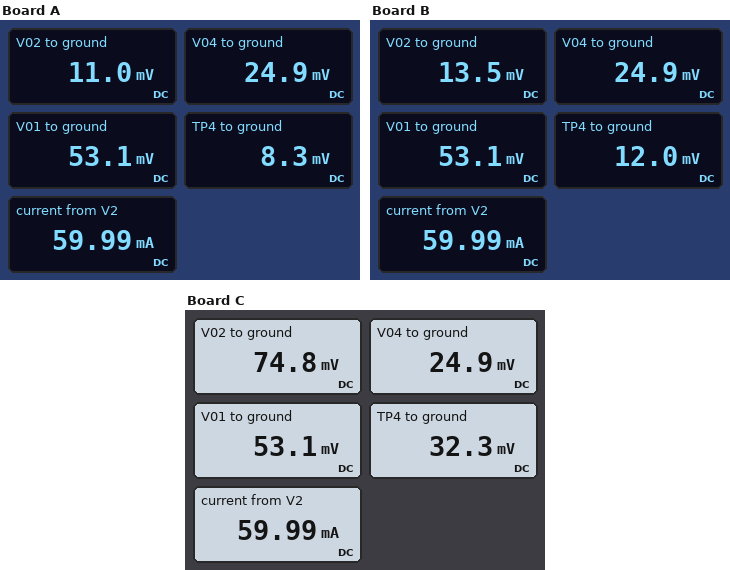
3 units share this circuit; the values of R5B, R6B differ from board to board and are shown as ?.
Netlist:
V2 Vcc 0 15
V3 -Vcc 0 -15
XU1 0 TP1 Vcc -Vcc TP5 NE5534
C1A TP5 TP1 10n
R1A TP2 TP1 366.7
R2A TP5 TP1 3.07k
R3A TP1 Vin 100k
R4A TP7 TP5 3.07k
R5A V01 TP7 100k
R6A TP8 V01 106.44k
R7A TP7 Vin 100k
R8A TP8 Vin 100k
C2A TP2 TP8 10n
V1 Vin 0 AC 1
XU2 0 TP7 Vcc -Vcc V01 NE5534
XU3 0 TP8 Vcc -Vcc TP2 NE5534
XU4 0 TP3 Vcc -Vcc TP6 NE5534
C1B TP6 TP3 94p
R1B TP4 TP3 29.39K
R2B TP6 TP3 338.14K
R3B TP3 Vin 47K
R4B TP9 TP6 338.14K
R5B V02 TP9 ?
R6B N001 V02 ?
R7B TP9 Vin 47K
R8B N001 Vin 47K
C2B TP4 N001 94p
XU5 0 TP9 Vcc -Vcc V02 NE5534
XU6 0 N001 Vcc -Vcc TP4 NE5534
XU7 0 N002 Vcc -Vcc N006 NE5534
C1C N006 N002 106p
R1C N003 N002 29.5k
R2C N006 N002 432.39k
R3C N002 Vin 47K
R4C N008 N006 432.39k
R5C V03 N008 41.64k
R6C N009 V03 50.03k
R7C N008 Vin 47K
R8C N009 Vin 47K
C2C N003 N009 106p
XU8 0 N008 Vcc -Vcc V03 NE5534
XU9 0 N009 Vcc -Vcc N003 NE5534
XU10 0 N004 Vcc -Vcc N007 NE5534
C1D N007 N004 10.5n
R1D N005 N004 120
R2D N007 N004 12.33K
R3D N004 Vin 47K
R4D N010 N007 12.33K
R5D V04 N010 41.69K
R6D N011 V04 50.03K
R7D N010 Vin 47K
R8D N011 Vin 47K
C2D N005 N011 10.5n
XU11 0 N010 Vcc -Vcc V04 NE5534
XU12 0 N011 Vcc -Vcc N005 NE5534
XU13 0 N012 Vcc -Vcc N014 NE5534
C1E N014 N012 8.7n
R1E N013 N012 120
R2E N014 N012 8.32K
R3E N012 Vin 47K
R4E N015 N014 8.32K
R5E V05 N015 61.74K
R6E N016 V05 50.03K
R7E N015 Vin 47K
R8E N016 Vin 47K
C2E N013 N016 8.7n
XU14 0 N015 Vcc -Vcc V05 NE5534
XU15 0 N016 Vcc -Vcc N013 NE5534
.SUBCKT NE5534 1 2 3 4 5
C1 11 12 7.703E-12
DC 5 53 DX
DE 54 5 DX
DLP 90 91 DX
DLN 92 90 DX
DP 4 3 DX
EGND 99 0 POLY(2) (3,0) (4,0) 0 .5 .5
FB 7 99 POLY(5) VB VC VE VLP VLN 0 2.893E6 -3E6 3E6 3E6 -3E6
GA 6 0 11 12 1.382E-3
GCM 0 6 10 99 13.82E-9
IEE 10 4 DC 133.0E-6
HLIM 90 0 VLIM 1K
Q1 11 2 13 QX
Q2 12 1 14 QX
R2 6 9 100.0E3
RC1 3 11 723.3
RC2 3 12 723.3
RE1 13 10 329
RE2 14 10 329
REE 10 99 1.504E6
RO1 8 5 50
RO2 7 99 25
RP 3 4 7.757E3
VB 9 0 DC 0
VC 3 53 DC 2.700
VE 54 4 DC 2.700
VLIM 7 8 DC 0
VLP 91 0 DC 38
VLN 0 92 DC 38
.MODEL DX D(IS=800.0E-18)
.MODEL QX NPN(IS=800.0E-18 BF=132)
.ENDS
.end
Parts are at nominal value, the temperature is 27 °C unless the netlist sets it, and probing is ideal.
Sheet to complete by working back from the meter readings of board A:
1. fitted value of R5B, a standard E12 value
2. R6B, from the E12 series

39 kΩ
22 kΩ
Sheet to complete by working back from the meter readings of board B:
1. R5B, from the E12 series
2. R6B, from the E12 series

33 kΩ
27 kΩ
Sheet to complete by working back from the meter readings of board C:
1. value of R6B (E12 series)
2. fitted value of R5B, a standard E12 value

150 kΩ
68 kΩ
